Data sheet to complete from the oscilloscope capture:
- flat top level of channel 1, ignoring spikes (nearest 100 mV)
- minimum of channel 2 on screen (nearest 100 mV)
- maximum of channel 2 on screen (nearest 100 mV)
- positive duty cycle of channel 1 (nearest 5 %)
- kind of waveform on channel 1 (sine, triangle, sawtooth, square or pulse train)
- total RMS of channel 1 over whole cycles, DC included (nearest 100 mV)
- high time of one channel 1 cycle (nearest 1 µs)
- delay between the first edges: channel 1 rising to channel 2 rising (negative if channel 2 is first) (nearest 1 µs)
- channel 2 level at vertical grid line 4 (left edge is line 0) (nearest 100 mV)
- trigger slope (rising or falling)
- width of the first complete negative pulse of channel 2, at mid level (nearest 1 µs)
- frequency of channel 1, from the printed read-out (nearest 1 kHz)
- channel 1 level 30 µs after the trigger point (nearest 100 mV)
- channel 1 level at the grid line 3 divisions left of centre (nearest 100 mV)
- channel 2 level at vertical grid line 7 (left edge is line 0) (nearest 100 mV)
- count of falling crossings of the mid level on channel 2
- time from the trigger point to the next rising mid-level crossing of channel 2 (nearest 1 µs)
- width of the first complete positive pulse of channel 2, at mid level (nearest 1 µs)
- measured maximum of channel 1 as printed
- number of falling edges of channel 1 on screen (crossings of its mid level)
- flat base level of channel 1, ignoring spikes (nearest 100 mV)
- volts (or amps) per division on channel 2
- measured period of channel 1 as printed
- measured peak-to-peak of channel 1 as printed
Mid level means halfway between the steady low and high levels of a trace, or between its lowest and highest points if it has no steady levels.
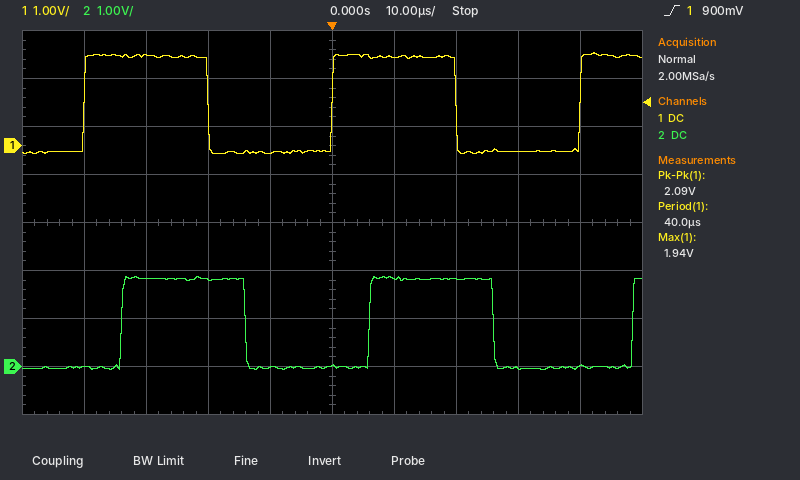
1.9 V
-100 mV
1.9 V
50 %
square
1.3 V
20 µs
+6 µs
0.0 V
rising
20 µs
25 kHz
-100 mV
1.9 V
1.8 V
2
6 µs
20 µs
1.94 V
2
-100 mV
1 V
40.0 µs
2.09 V
